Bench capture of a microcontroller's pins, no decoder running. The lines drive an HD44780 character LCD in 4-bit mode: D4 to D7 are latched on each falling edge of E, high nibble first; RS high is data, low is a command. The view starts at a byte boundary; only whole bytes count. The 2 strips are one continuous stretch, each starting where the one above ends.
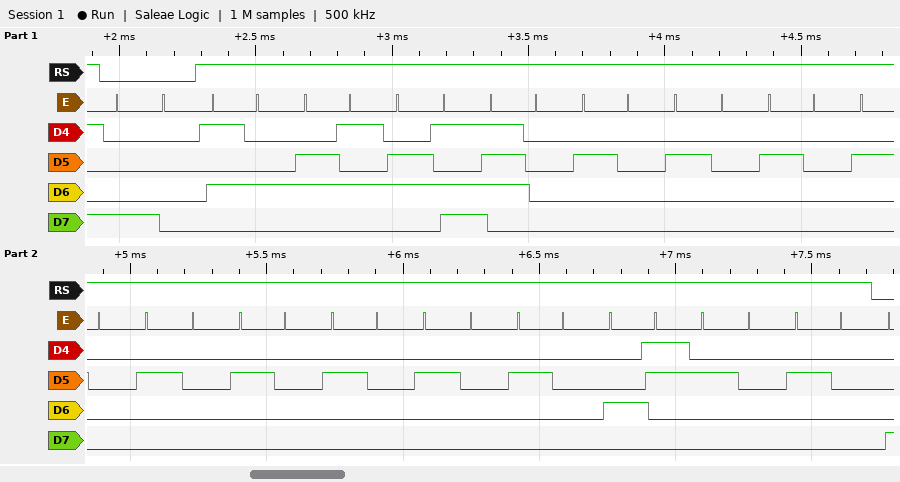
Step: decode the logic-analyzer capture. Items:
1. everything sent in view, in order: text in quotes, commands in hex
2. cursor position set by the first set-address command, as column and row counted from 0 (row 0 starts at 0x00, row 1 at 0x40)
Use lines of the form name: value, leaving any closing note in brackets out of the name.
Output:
everything sent in view, in order: text in quotes, commands in hex: 0x80 "Temp         C  "
cursor position set by the first set-address command, as column and row counted from 0: column 0, row 0
